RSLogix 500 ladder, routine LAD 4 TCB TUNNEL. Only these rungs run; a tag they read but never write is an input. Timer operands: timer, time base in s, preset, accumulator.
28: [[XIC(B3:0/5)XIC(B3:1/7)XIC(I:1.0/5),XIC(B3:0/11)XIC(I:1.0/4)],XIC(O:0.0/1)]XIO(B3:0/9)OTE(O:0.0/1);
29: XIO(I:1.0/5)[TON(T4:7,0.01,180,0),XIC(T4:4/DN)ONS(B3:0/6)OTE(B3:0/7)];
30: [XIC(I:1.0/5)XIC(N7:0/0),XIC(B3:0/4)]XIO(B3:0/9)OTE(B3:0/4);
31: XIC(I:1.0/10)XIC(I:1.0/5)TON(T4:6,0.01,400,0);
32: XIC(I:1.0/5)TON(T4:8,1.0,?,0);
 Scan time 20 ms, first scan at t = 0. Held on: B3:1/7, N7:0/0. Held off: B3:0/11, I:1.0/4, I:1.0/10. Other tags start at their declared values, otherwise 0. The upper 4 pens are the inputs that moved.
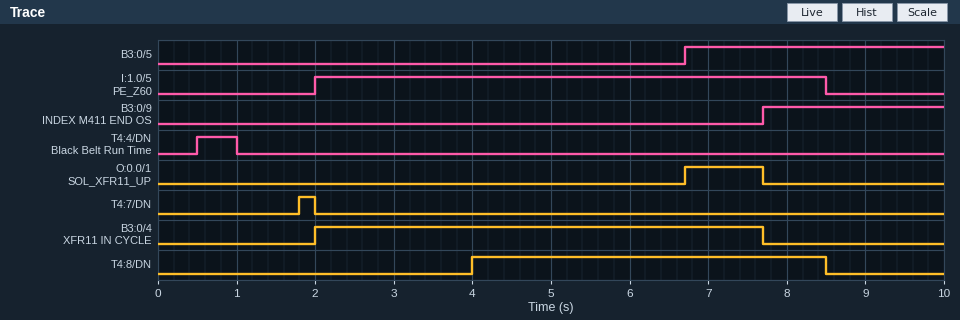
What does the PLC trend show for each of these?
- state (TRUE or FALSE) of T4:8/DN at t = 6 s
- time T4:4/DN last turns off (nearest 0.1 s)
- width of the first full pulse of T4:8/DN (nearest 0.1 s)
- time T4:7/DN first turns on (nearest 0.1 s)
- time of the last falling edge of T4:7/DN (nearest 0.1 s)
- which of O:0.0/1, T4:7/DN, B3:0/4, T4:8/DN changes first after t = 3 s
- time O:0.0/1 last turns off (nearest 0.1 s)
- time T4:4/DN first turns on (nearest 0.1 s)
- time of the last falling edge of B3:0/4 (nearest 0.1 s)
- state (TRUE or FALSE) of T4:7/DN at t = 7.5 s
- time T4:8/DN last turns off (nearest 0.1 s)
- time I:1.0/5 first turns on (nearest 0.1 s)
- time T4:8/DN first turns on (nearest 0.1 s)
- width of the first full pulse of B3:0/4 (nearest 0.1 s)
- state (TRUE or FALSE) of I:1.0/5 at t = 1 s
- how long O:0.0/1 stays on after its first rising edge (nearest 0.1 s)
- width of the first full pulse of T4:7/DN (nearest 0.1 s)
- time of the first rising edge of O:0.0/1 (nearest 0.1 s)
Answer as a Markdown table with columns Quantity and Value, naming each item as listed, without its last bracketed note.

| Quantity | Value |
|---|---|
| state (TRUE or FALSE) of T4:8/DN at t = 6 s | TRUE |
| time T4:4/DN last turns off | 1.0 s |
| width of the first full pulse of T4:8/DN | 4.5 s |
| time T4:7/DN first turns on | 1.8 s |
| time of the last falling edge of T4:7/DN | 2.0 s |
| which of O:0.0/1, T4:7/DN, B3:0/4, T4:8/DN changes first after t = 3 s | T4:8/DN |
| time O:0.0/1 last turns off | 7.7 s |
| time T4:4/DN first turns on | 0.5 s |
| time of the last falling edge of B3:0/4 | 7.7 s |
| state (TRUE or FALSE) of T4:7/DN at t = 7.5 s | FALSE |
| time T4:8/DN last turns off | 8.5 s |
| time I:1.0/5 first turns on | 2.0 s |
| time T4:8/DN first turns on | 4.0 s |
| width of the first full pulse of B3:0/4 | 5.7 s |
| state (TRUE or FALSE) of I:1.0/5 at t = 1 s | FALSE |
| how long O:0.0/1 stays on after its first rising edge | 1.0 s |
| width of the first full pulse of T4:7/DN | 0.2 s |
| time of the first rising edge of O:0.0/1 | 6.7 s |
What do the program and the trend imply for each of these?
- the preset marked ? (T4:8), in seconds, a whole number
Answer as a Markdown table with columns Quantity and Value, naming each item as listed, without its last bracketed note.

| Quantity | Value |
|---|---|
| the preset marked ? (T4:8), in seconds, a whole number | 2 s |
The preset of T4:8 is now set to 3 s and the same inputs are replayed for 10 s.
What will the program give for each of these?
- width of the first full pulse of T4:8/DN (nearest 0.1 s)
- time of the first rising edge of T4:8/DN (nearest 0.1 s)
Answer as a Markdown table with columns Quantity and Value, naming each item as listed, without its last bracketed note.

| Quantity | Value |
|---|---|
| width of the first full pulse of T4:8/DN | 3.5 s |
| time of the first rising edge of T4:8/DN | 5.0 s |
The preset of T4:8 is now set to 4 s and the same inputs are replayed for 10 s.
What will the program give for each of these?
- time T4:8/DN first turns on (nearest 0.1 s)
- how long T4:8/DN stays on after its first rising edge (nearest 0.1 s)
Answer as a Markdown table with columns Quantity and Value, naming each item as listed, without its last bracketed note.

| Quantity | Value |
|---|---|
| time T4:8/DN first turns on | 6.0 s |
| how long T4:8/DN stays on after its first rising edge | 2.5 s |
